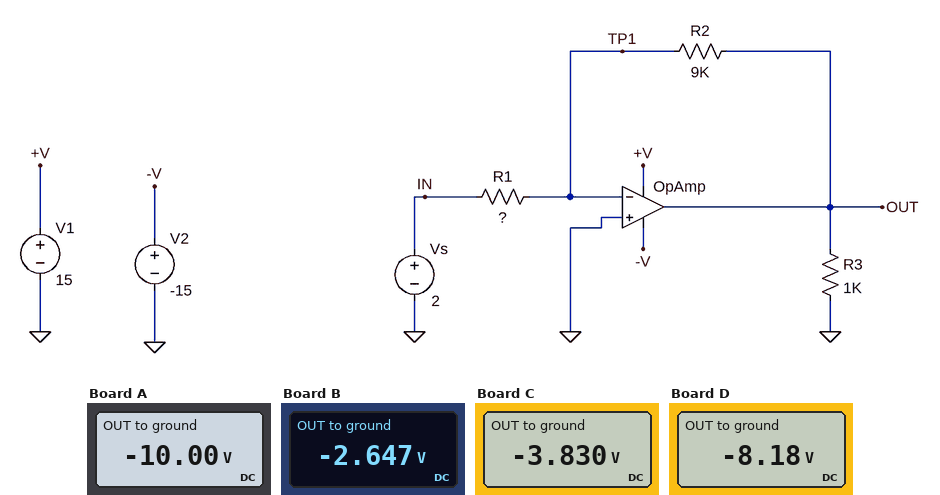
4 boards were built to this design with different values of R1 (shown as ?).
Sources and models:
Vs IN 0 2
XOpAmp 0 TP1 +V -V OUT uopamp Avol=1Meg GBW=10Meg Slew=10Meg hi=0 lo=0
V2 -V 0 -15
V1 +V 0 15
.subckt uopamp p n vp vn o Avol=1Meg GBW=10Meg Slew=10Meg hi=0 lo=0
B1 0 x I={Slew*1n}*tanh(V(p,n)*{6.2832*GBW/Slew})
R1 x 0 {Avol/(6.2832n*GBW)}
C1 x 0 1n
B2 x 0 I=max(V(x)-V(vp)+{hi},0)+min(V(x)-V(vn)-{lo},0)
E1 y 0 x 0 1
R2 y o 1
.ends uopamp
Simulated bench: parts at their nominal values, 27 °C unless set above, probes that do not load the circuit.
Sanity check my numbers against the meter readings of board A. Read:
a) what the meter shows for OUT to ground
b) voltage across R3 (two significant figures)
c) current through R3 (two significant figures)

-10.00 V
10 V
10 mA
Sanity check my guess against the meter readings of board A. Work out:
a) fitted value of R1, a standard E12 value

1.8 kΩ
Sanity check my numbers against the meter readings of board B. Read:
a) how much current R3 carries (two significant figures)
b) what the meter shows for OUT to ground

2.6 mA
-2.647 V
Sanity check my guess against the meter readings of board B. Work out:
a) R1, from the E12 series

6.8 kΩ
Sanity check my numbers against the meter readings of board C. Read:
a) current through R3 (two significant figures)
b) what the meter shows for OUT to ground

3.8 mA
-3.830 V
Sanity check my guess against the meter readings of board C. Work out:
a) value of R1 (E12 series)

4.7 kΩ
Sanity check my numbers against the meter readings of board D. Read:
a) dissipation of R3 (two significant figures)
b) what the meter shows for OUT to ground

67 mW
-8.18 V
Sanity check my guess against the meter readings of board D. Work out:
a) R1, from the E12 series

2.2 kΩ
